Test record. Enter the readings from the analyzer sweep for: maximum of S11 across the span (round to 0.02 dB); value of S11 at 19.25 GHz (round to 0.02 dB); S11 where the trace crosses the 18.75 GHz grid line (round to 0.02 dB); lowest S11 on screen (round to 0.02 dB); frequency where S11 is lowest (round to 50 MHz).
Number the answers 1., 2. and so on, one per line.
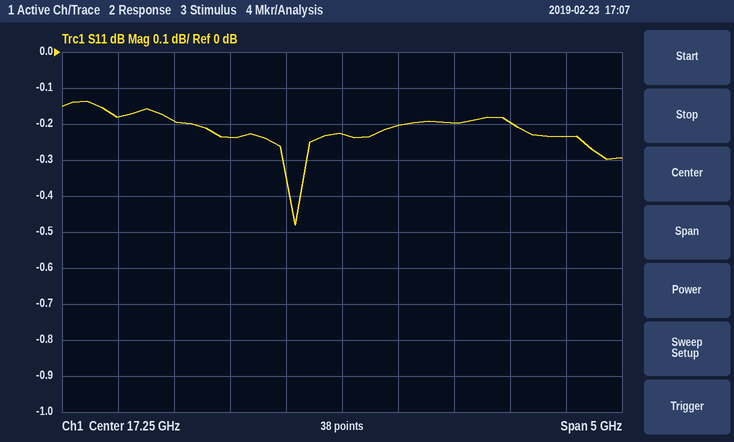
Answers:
1. -0.14 dB
2. -0.24 dB
3. -0.20 dB
4. -0.48 dB
5. 16.85 GHz
